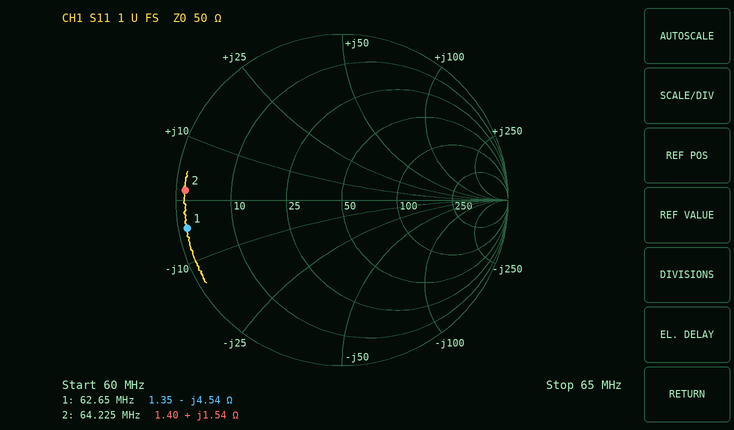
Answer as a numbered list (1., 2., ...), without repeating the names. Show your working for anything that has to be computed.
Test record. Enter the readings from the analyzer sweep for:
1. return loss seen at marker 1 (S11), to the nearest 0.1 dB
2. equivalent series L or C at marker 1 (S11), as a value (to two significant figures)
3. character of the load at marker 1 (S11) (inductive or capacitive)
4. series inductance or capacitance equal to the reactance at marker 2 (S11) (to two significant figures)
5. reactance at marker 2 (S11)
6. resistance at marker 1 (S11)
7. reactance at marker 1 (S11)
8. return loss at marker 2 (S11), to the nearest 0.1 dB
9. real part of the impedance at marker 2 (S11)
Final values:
1. 0.5 dB
2. C = 1/(2π × 62.65 MHz × 4.54 Ω) ≈ 560 pF
3. capacitive
4. L = 1.54 Ω/(2π × 64.225 MHz) ≈ 3.8 nH
5. +1.54 Ω
6. 1.35 Ω
7. -4.54 Ω
8. 0.5 dB
9. 1.40 Ω
